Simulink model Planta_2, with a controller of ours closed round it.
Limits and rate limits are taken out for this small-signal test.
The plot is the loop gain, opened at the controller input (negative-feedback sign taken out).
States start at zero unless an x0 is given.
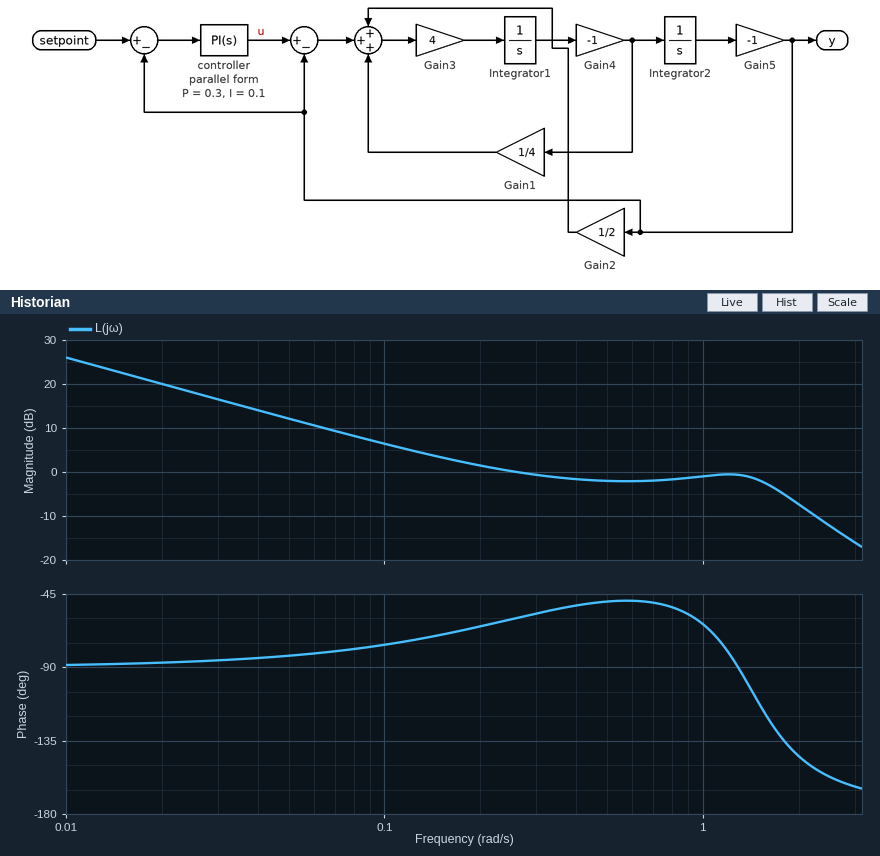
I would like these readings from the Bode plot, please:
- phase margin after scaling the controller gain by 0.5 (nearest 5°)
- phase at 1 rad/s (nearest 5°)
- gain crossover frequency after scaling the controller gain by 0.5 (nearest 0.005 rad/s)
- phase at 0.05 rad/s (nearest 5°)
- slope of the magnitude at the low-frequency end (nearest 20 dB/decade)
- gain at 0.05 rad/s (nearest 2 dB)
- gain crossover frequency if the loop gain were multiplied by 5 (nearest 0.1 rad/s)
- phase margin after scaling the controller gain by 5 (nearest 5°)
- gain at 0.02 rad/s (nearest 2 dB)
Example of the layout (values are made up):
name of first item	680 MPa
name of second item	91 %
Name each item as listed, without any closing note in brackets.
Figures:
phase margin after scaling the controller gain by 0.5	105°
phase at 1 rad/s	-65°
gain crossover frequency after scaling the controller gain by 0.5	0.105 rad/s
phase at 0.05 rad/s	-85°
slope of the magnitude at the low-frequency end	-20 dB/decade
gain at 0.05 rad/s	12 dB
gain crossover frequency if the loop gain were multiplied by 5	2.7 rad/s
phase margin after scaling the controller gain by 5	20°
gain at 0.02 rad/s	20 dB
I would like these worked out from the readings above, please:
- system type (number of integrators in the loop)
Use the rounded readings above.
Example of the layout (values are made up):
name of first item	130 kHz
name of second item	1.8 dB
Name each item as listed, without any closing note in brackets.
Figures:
system type	1
